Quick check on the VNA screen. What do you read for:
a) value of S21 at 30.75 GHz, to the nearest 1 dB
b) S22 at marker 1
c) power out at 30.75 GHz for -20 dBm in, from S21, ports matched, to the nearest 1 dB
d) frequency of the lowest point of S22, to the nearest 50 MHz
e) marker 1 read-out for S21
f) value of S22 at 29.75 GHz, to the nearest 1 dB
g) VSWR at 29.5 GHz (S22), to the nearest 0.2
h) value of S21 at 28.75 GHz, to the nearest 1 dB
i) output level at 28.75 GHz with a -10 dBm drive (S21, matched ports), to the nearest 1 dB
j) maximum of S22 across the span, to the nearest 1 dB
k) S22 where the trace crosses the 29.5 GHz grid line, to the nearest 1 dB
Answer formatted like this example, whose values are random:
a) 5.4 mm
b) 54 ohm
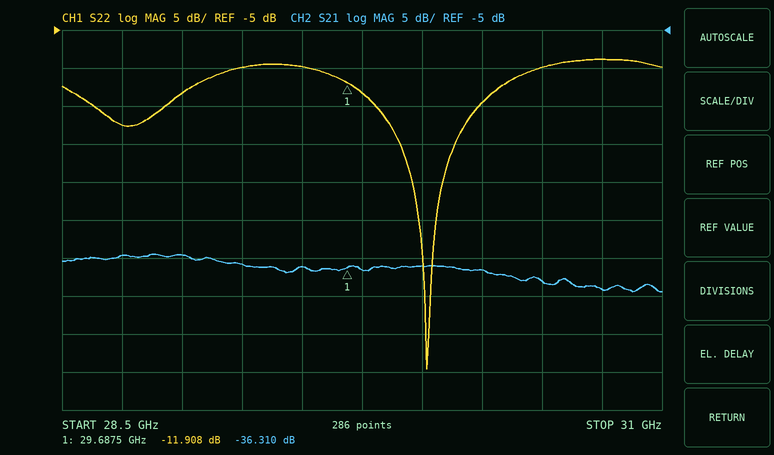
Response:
a) -39 dB
b) -11.908 dB
c) -59 dBm
d) 30.00 GHz
e) -36.310 dB
f) -13 dB
g) 2.0
h) -35 dB
i) -45 dBm
j) -9 dB
k) -10 dB
